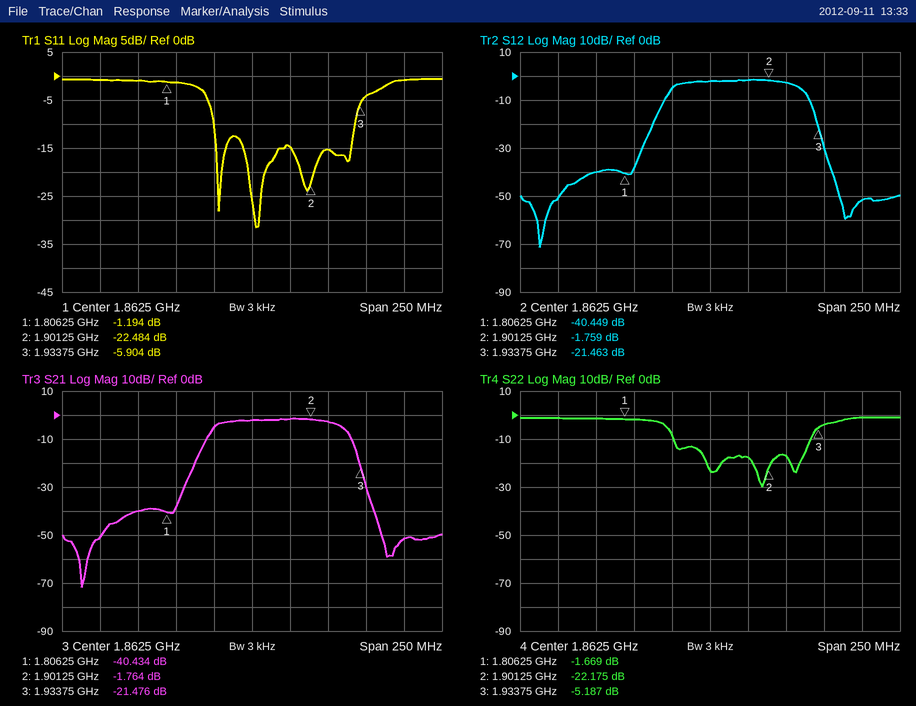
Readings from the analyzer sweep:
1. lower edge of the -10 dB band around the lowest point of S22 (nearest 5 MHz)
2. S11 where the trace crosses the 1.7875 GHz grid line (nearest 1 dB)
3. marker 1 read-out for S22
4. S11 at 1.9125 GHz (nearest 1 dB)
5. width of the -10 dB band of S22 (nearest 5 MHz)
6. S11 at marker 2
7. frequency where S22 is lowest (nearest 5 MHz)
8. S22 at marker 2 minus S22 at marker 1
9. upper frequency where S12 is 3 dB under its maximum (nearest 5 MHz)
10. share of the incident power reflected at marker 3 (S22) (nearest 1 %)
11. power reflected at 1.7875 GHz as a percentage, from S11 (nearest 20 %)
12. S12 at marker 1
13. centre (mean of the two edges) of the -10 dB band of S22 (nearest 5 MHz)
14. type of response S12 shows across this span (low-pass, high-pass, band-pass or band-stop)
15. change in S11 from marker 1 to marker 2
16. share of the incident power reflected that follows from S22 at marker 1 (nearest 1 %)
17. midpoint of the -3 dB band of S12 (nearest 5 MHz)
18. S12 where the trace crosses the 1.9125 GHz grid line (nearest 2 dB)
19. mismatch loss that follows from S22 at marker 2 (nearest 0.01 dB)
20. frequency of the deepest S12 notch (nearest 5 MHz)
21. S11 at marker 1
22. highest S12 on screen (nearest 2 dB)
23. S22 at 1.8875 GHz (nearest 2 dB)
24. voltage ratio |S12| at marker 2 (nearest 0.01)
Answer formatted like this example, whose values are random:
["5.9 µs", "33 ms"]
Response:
["1.840 GHz", "-1 dB", "-1.669 dB", "-15 dB", "90 MHz", "-22.484 dB", "1.895 GHz", "-20.506 dB", "1.920 GHz", "30 %", "80 %", "-40.449 dB", "1.885 GHz", "band-pass", "-21.290 dB", "68 %", "1.880 GHz", "-2 dB", "0.03 dB", "1.750 GHz", "-1.194 dB", "-2 dB", "-18 dB", "0.82"]
